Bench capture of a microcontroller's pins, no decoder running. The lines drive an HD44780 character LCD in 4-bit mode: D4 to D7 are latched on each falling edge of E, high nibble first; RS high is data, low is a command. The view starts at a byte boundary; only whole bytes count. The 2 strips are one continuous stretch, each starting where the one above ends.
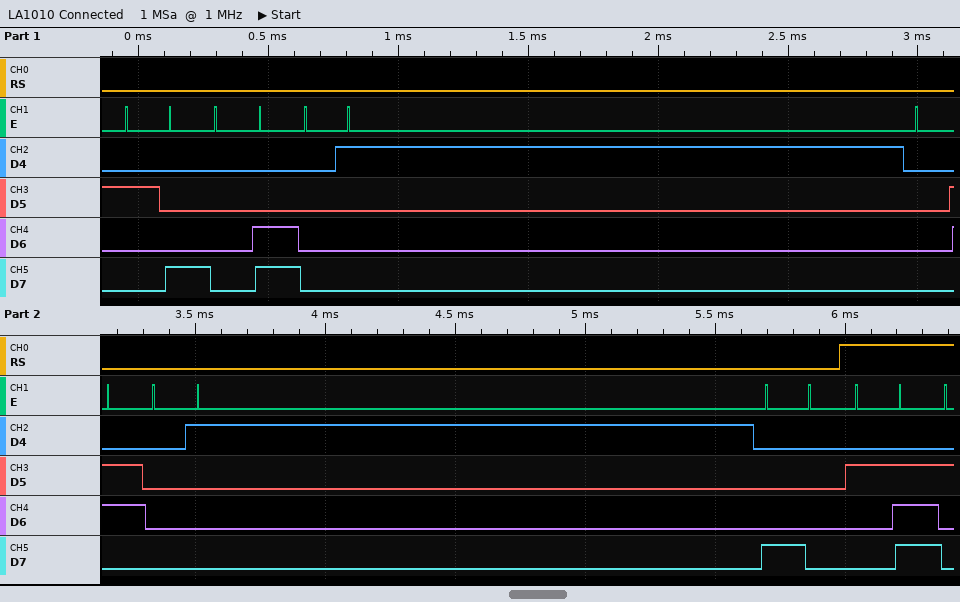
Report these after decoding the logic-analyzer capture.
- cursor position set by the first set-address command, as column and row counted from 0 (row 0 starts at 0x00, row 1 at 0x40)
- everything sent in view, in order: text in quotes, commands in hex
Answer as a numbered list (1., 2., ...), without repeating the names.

1. column 0, row 0
2. 0x28 0x0C 0x01 0x06 0x01 0x80 "."
